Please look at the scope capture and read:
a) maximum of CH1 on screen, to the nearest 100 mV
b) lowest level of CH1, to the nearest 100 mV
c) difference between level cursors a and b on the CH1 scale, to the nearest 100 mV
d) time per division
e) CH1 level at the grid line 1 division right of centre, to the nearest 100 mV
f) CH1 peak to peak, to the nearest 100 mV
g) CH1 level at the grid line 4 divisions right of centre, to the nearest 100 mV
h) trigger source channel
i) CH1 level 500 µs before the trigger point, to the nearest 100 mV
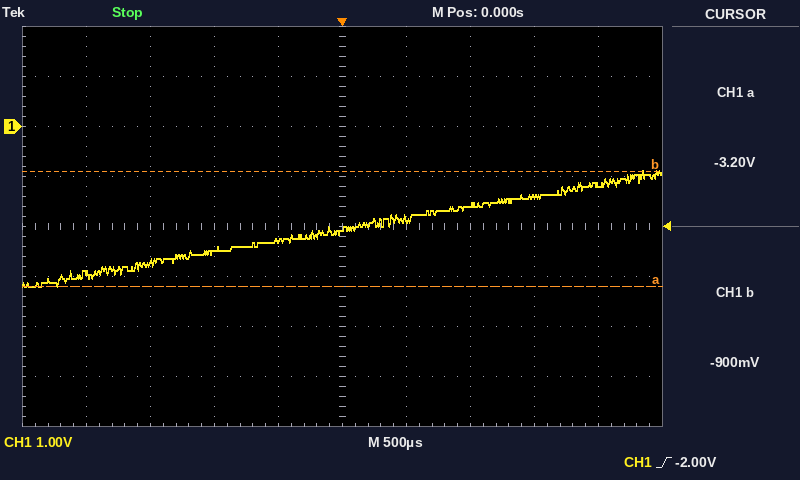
-900 mV
-3.2 V
2.3 V
500 µs
-1.8 V
2.3 V
-1.2 V
CH1
-2.3 V
